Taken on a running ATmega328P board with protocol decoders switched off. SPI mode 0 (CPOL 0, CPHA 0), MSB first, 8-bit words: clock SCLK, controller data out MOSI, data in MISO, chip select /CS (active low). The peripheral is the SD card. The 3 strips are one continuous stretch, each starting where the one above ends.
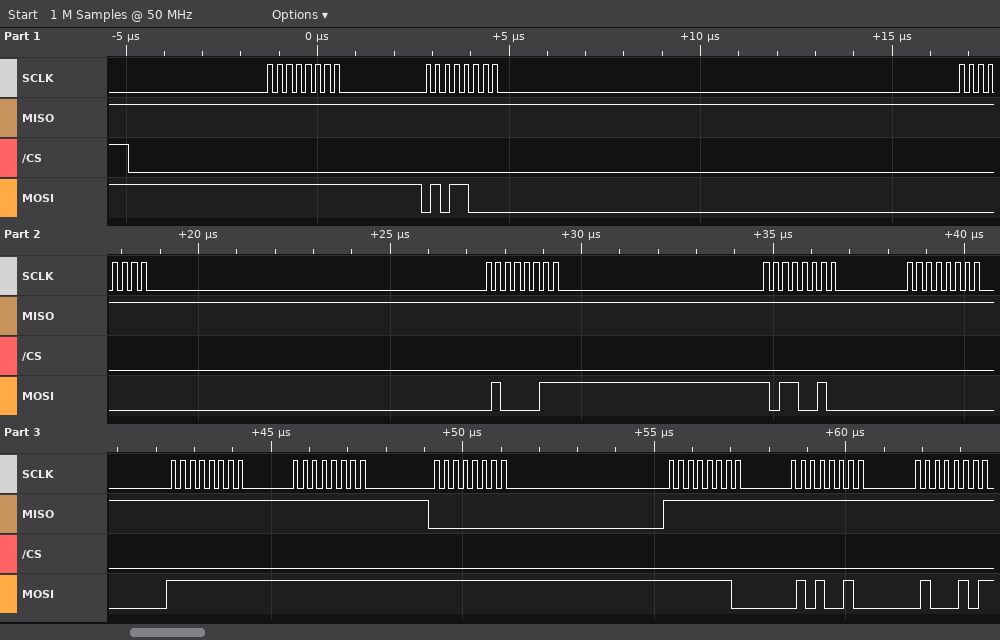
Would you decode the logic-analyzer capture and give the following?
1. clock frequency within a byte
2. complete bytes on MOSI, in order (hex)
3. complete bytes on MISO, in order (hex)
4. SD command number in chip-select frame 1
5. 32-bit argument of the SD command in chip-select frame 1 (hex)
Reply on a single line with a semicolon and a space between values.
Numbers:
4 MHz; 0xFF 0x58 0x00 0x43 0xB2 0x00 0xFF 0xFF 0xFF 0xFE 0x52 0x45; 0xFF 0xFF 0xFF 0xFF 0xFF 0xFF 0xFF 0xFF 0x00 0xFF 0xFF 0xFF; CMD24; 0x0043B200
